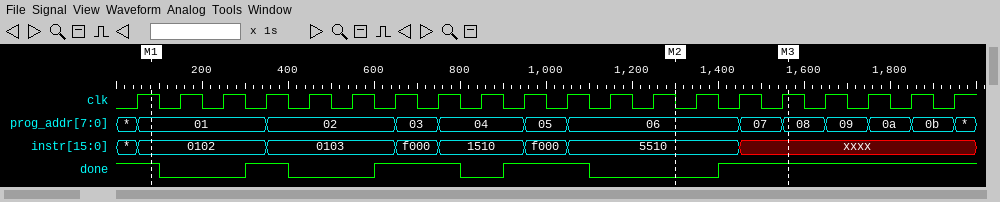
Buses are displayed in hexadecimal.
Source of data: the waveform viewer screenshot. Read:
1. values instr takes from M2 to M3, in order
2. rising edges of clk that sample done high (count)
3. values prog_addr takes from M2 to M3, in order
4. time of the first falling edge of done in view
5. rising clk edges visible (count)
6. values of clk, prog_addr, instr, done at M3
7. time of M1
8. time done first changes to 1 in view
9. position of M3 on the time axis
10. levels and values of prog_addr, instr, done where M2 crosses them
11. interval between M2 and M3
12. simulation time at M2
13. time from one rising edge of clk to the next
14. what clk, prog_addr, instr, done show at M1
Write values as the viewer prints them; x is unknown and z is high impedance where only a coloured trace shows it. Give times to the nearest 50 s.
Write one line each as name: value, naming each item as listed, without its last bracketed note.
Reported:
values instr takes from M2 to M3, in order: 5510, xxxx
rising edges of clk that sample done high: 12
values prog_addr takes from M2 to M3, in order: 06, 07, 08
time of the first falling edge of done in view: 100 s
rising clk edges visible: 20
values of clk, prog_addr, instr, done at M3: clk=1, prog_addr=08, instr=xxxx, done=1
time of M1: 100 s
time done first changes to 1 in view: 300 s
position of M3 on the time axis: 1550 s
levels and values of prog_addr, instr, done where M2 crosses them: prog_addr=06, instr=5510, done=0
interval between M2 and M3: 250 s
simulation time at M2: 1300 s
time from one rising edge of clk to the next: 100 s
what clk, prog_addr, instr, done show at M1: clk=1, prog_addr=01, instr=0102, done=1
